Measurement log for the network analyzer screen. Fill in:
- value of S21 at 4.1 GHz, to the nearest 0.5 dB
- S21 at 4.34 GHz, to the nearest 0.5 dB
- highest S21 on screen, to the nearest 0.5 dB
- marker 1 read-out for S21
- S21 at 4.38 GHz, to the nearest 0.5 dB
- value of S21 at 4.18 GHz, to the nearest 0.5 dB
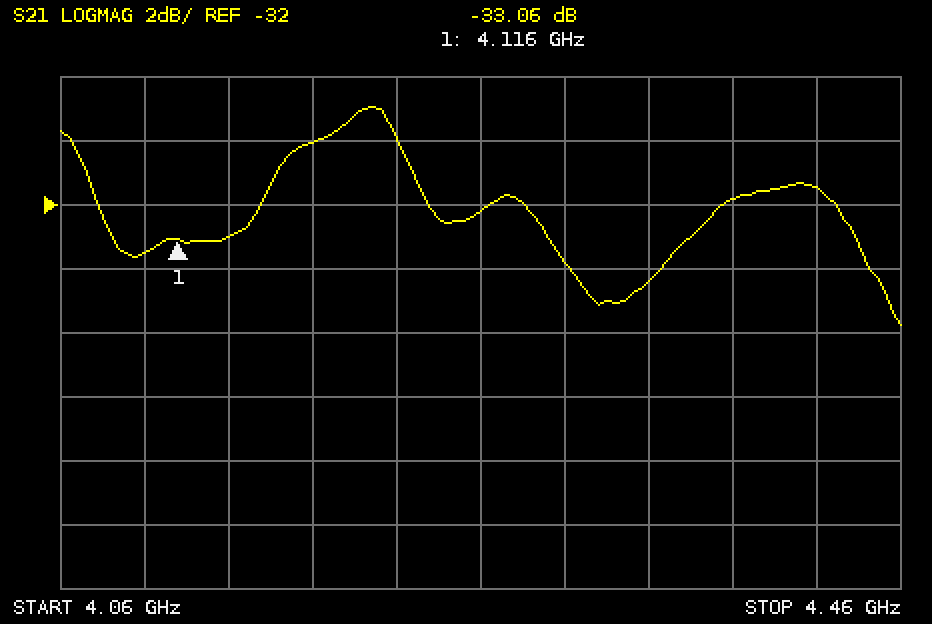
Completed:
-33.5 dB
-34.5 dB
-29.0 dB
-33.06 dB
-32.0 dB
-30.0 dB
